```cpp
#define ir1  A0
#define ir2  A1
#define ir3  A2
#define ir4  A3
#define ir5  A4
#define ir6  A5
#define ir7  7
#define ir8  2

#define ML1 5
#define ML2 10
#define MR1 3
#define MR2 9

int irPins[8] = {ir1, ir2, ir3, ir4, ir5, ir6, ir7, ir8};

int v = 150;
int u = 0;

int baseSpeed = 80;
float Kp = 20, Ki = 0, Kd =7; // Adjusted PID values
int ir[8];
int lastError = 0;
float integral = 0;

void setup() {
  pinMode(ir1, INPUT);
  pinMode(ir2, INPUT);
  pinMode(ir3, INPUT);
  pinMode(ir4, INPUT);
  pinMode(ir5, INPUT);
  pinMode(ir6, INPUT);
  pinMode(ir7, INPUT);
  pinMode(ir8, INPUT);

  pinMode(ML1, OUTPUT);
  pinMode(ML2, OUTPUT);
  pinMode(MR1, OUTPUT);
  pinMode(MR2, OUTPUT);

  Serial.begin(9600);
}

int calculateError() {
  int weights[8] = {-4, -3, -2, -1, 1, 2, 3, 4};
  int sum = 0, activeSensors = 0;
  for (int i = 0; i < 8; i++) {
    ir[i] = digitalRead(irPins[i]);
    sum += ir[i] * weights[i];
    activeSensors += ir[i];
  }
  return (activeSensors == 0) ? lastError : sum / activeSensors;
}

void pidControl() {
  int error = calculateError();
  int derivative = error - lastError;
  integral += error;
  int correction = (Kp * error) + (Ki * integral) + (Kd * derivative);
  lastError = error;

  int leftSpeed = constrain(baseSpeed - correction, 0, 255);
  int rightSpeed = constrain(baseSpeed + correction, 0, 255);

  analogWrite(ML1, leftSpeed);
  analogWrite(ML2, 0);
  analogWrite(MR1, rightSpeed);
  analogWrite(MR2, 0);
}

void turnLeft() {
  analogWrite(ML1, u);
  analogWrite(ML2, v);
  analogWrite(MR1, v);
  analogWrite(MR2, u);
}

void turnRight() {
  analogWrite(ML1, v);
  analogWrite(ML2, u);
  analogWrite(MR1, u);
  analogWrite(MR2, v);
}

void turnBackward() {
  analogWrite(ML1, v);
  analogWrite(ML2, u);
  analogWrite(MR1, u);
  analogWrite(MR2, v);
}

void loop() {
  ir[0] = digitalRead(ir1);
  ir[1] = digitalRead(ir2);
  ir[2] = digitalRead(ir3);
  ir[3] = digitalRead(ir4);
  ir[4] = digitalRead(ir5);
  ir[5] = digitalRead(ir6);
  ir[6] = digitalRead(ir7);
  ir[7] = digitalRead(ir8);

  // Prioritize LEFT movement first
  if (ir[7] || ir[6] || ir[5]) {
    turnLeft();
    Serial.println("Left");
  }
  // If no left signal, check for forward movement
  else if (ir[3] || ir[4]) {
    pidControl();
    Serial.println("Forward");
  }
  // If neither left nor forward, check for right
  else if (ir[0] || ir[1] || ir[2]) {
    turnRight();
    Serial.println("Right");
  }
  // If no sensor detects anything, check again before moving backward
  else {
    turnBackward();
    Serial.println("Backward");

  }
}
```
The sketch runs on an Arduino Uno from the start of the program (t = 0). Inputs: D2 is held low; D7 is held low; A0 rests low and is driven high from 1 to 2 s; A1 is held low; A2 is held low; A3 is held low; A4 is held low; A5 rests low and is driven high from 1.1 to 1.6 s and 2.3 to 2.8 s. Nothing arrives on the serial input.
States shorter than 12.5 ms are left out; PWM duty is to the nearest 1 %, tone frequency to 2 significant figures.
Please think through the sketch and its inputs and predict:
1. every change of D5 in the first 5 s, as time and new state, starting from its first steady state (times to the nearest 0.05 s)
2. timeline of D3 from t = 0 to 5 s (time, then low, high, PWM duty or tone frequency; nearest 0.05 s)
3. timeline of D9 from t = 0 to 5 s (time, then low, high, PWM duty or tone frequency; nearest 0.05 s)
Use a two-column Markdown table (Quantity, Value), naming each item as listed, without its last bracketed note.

| Quantity | Value |
|---|---|
| every change of D5 in the first 5 s, as time and new state, starting from its first steady state | 0 s PWM 59 %; 1.1 s low; 1.6 s PWM 59 %; 2.3 s low; 2.8 s PWM 59 % |
| timeline of D3 from t = 0 to 5 s | 0 s low; 1.1 s PWM 59 %; 1.6 s low; 2.3 s PWM 59 %; 2.8 s low |
| timeline of D9 from t = 0 to 5 s | 0 s PWM 59 %; 1.1 s low; 1.6 s PWM 59 %; 2.3 s low; 2.8 s PWM 59 % |
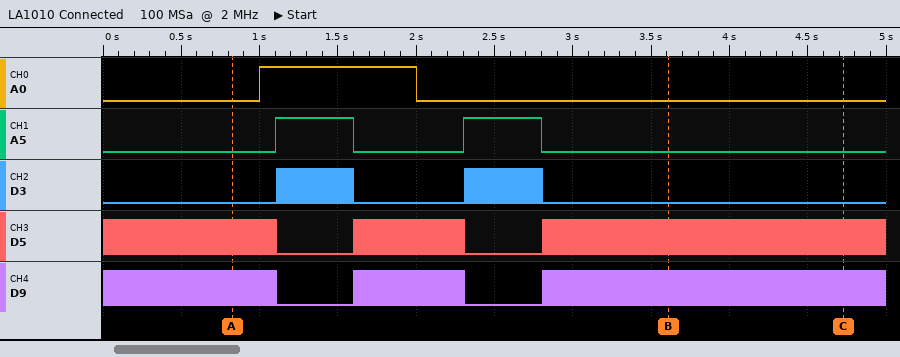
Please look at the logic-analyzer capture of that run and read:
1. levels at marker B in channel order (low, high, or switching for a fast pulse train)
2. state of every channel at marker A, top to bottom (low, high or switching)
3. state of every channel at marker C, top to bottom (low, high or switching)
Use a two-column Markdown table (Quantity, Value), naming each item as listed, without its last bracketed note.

| Quantity | Value |
|---|---|
| levels at marker B in channel order | A0 low, A5 low, D3 low, D5 switching, D9 switching |
| state of every channel at marker A, top to bottom | A0 low, A5 low, D3 low, D5 switching, D9 switching |
| state of every channel at marker C, top to bottom | A0 low, A5 low, D3 low, D5 switching, D9 switching |
